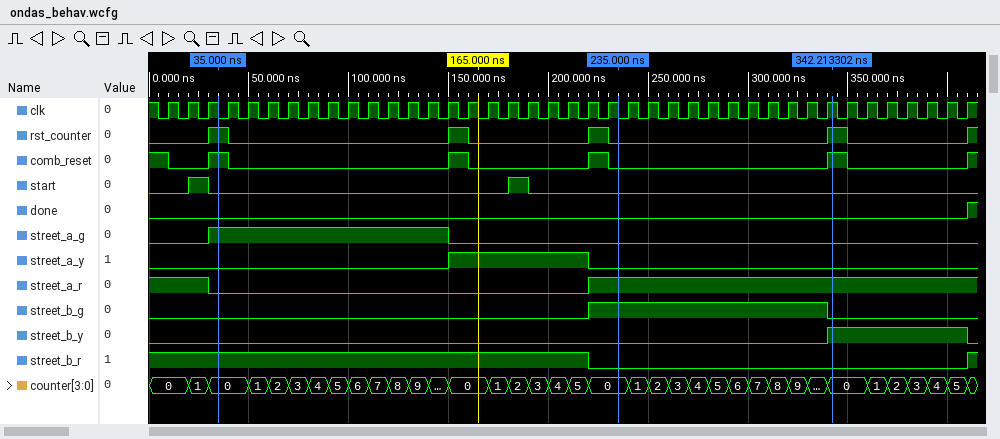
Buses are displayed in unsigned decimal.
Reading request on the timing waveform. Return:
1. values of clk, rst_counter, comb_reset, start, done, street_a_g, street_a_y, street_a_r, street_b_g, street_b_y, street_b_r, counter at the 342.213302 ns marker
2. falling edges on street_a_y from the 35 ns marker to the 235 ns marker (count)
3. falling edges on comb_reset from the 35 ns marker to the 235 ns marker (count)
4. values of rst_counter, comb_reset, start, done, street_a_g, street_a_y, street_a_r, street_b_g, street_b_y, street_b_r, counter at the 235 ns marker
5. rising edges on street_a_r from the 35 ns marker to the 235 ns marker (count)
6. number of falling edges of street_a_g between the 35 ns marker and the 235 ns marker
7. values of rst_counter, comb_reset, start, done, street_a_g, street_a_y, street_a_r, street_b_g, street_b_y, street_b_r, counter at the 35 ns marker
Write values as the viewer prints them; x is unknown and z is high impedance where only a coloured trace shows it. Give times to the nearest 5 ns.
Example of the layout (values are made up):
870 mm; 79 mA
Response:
clk=1, rst_counter=1, comb_reset=1, start=0, done=0, street_a_g=0, street_a_y=0, street_a_r=1, street_b_g=0, street_b_y=1, street_b_r=0, counter=0; 1; 3; rst_counter=0, comb_reset=0, start=0, done=0, street_a_g=0, street_a_y=0, street_a_r=1, street_b_g=1, street_b_y=0, street_b_r=0, counter=0; 1; 1; rst_counter=1, comb_reset=1, start=0, done=0, street_a_g=1, street_a_y=0, street_a_r=0, street_b_g=0, street_b_y=0, street_b_r=1, counter=0
